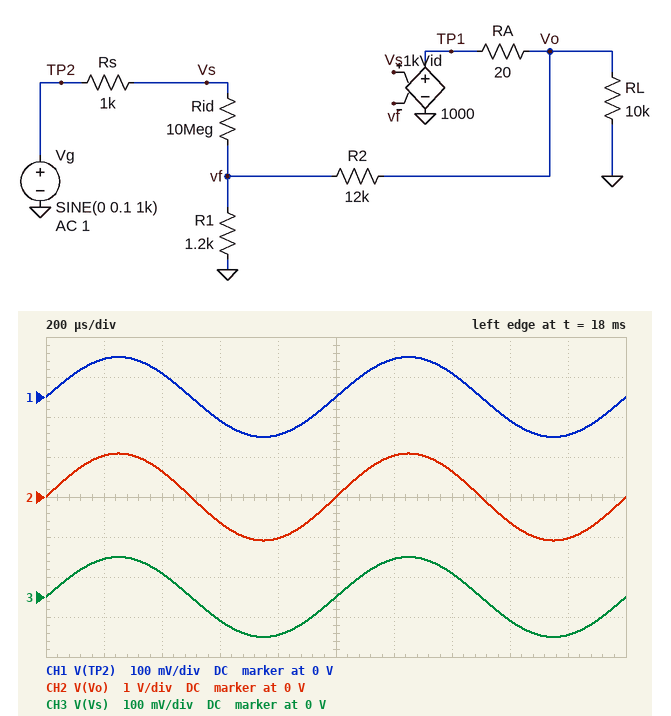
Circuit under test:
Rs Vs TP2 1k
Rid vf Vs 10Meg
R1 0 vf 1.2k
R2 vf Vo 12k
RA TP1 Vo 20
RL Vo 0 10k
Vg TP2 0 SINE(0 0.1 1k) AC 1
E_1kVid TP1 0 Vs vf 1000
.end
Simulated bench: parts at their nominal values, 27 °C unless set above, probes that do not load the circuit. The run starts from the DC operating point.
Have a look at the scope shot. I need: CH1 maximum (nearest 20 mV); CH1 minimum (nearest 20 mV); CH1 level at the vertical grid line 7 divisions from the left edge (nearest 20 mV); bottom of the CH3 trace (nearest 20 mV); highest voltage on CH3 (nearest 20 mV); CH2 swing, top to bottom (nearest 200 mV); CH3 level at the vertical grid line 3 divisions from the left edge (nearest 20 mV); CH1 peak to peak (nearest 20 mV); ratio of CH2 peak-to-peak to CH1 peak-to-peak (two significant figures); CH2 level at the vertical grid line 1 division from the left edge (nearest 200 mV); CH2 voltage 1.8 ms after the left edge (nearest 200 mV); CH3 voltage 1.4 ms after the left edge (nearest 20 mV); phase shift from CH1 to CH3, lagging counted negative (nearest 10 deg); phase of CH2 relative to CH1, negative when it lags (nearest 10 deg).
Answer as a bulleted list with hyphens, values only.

- 100 mV
- -100 mV
- 60 mV
- -100 mV
- 100 mV
- 2.2 V
- -60 mV
- 200 mV
- 11
- 1.0 V
- -1.0 V
- 60 mV
- 0 deg
- 0 deg
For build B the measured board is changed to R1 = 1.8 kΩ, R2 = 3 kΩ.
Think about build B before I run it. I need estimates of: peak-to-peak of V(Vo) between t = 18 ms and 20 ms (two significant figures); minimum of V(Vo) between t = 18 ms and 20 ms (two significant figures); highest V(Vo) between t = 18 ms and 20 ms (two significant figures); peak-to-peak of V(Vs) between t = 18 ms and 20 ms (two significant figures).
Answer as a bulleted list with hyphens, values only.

- 530 mV
- -270 mV
- 270 mV
- 200 mV
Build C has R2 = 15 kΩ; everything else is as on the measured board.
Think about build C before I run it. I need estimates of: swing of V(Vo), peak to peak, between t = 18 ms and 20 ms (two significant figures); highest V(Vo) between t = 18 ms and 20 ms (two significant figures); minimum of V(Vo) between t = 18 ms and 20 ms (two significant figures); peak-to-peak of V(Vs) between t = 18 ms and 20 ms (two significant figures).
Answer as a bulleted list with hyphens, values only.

- 2.7 V
- 1.3 V
- -1.3 V
- 200 mV
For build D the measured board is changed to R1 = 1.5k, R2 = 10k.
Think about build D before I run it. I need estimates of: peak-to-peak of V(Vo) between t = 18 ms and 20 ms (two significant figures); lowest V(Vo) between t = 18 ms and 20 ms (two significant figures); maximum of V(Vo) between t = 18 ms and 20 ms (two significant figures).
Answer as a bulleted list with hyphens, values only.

- 1.5 V
- -760 mV
- 760 mV
